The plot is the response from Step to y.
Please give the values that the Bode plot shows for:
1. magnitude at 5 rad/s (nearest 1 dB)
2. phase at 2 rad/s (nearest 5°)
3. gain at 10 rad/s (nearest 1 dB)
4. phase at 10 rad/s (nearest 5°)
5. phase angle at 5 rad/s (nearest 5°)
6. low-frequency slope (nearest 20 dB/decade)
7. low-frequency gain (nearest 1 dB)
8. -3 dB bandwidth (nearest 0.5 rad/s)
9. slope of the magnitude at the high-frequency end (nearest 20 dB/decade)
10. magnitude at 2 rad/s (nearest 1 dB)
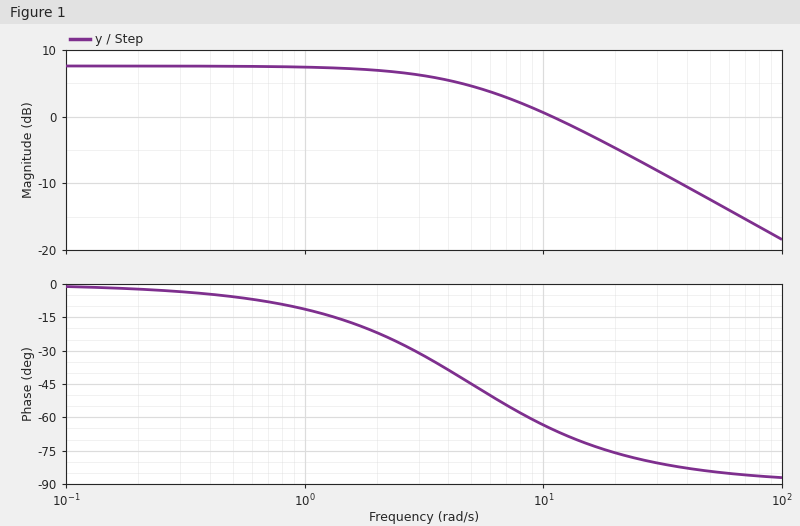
5 dB
-20°
1 dB
-65°
-45°
0 dB/decade
8 dB
5.0 rad/s
-20 dB/decade
7 dB
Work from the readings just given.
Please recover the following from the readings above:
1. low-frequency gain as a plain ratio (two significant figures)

2.5
